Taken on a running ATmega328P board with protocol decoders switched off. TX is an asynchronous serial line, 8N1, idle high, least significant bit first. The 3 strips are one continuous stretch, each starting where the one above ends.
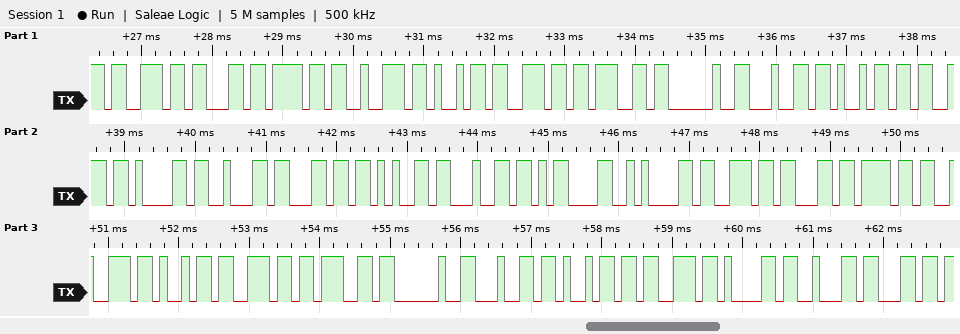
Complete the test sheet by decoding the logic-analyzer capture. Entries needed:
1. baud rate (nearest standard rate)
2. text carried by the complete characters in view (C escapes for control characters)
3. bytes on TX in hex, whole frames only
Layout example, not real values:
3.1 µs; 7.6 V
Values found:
9600 baud; "scoring disabled\r\nscoring disabl"; 0x73 0x63 0x6F 0x72 0x69 0x6E 0x67 0x20 0x64 0x69 0x73 0x61 0x62 0x6C 0x65 0x64 0x0D 0x0A 0x73 0x63 0x6F 0x72 0x69 0x6E 0x67 0x20 0x64 0x69 0x73 0x61 0x62 0x6C
